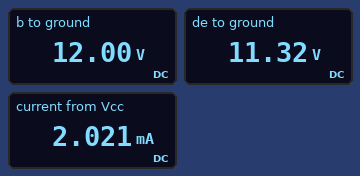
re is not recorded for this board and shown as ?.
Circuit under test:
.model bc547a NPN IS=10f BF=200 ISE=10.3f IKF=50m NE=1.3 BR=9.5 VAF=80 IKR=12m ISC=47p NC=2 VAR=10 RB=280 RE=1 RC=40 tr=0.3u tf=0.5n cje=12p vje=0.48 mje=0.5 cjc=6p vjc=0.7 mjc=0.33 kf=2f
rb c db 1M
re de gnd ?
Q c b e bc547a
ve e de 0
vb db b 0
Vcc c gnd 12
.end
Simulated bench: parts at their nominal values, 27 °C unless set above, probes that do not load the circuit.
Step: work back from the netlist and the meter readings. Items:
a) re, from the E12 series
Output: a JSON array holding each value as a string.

["5.6 kΩ"]
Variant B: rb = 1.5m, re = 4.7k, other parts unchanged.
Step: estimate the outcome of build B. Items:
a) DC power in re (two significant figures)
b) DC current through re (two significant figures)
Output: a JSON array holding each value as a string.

["27 mW", "2.4 mA"]
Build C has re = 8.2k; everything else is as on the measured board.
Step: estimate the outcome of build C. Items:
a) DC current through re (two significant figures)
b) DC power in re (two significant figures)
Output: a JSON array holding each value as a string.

["1.4 mA", "16 mW"]
